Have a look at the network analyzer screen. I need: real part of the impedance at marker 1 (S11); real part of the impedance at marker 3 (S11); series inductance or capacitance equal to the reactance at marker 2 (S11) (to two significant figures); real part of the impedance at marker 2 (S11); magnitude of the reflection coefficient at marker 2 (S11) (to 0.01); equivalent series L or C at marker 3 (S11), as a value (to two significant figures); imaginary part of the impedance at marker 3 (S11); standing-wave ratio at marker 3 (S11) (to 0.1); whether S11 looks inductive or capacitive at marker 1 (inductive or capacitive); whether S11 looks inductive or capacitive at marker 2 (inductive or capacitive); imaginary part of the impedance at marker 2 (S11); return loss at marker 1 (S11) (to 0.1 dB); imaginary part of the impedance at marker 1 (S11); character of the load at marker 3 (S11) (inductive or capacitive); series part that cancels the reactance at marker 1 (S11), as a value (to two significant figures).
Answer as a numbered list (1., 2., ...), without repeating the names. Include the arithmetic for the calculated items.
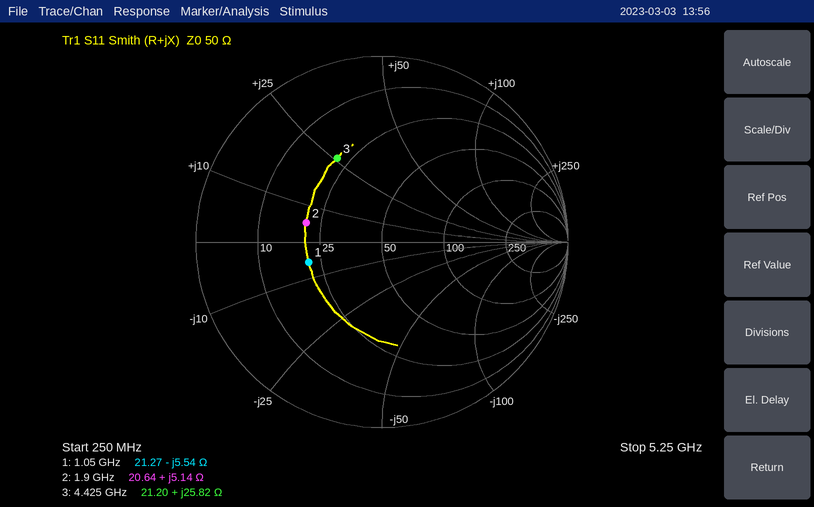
1. 21.27 Ω
2. 21.20 Ω
3. L = 5.14 Ω/(2π × 1.9 GHz) ≈ 431 pH, so 430 pH to two significant figures
4. 20.64 Ω
5. 0.42
6. L = 25.82 Ω/(2π × 4.425 GHz) ≈ 929 pH, so 930 pH to two significant figures
7. +25.82 Ω
8. 3.1
9. capacitive
10. inductive
11. +5.14 Ω
12. 7.8 dB
13. -5.54 Ω
14. inductive
15. L = 5.54 Ω/(2π × 1.05 GHz) ≈ 840 pH
